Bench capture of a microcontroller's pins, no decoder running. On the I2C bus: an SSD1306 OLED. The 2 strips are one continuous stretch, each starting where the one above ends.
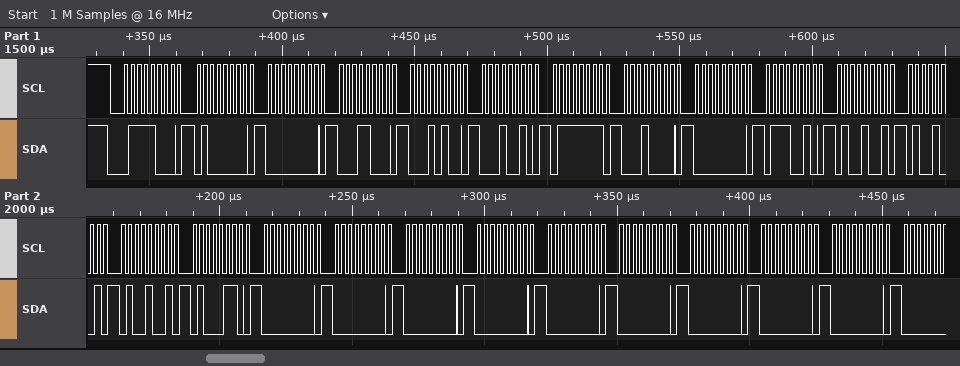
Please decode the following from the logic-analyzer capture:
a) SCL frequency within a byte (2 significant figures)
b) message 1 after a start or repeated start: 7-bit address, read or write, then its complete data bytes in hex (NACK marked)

400 kHz
0x3C write: 40 00 18 14 12 7F 10 00 72 49 49 49 46 00 00 00 00 00 00 00 00 00
